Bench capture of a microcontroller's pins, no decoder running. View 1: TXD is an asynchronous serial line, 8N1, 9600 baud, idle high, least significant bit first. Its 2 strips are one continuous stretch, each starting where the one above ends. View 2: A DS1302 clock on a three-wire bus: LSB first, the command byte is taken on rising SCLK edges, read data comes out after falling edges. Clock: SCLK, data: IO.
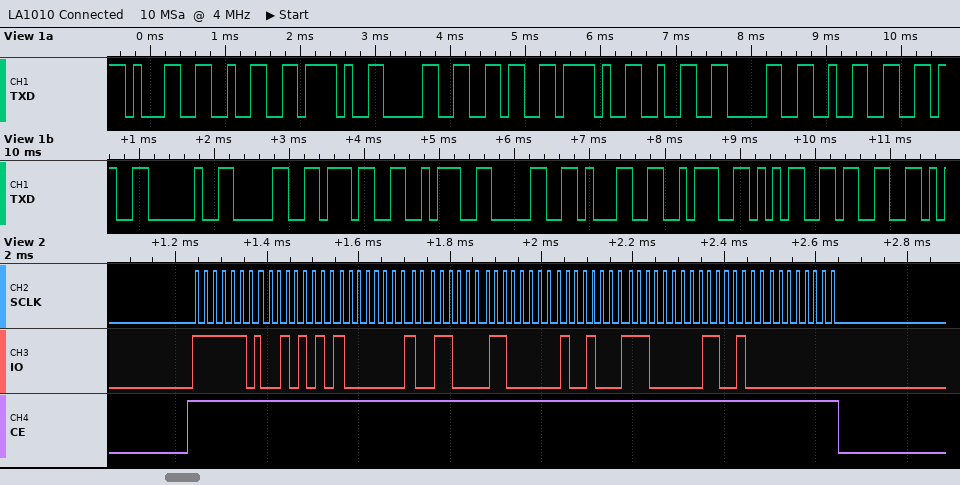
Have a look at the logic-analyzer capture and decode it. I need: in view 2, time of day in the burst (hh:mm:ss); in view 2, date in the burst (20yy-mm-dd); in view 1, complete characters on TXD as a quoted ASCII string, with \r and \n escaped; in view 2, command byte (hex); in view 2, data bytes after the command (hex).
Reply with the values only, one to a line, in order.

19:01:54
2026-12-06
"12/06/2026 07:01:53"
0xBF
54 01 19 06 12 07 26 00
